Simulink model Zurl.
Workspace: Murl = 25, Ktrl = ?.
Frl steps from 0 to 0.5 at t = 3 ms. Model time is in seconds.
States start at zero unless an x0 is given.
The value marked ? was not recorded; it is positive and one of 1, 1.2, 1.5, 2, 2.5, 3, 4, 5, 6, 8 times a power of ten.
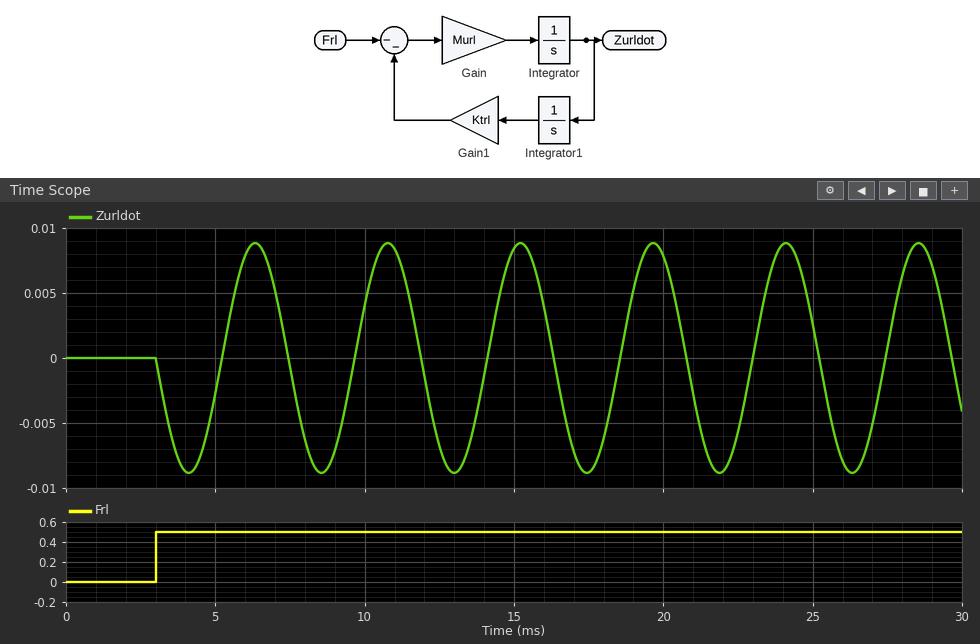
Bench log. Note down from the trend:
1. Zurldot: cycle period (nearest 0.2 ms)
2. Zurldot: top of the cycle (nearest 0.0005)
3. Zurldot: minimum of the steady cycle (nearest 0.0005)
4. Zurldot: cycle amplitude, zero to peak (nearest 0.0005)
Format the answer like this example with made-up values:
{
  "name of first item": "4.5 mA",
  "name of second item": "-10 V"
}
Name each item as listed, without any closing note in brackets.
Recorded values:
{
  "Zurldot: cycle period": "4.4 ms",
  "Zurldot: top of the cycle": "0.0090",
  "Zurldot: minimum of the steady cycle": "-0.0090",
  "Zurldot: cycle amplitude, zero to peak": "0.0090"
}
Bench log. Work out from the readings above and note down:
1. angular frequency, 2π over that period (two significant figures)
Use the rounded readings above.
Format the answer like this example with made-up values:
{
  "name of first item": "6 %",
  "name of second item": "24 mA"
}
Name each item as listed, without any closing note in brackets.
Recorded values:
{
  "angular frequency, 2π over that period": "1.4 rad/ms"
}
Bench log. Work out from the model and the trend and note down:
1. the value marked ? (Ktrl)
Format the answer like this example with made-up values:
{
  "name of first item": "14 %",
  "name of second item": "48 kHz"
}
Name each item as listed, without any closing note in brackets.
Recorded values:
{
  "the value marked ?": "80000"
}
